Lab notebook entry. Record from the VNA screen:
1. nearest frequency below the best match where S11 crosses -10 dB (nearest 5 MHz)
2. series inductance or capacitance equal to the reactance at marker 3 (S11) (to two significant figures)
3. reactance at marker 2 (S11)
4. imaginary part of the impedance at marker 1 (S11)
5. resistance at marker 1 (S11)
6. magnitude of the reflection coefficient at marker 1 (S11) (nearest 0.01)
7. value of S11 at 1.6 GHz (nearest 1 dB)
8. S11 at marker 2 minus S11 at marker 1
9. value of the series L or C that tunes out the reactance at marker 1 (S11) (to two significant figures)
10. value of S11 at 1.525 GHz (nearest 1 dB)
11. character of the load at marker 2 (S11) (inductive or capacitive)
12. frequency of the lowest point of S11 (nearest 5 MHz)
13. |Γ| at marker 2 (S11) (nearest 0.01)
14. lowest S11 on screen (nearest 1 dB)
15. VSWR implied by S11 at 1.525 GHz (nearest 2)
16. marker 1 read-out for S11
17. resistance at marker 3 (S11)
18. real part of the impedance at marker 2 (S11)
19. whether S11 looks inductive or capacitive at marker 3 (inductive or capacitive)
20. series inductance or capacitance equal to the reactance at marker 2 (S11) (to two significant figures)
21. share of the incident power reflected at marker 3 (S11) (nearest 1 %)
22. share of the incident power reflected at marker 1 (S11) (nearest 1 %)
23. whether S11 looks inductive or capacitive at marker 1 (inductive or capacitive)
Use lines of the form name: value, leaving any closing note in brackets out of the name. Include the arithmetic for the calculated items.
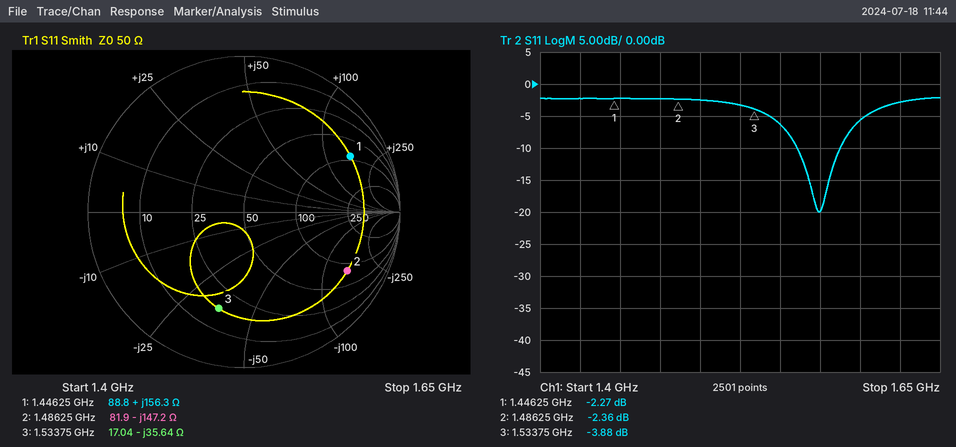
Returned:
nearest frequency below the best match where S11 crosses -10 dB: 1.560 GHz
series inductance or capacitance equal to the reactance at marker 3 (S11): C = 1/(2π × 1.53375 GHz × 35.64 Ω) ≈ 2.9 pF
reactance at marker 2: -147.2 Ω
imaginary part of the impedance at marker 1: +156.3 Ω
resistance at marker 1: 88.8 Ω
magnitude of the reflection coefficient at marker 1 (S11): 0.77
value of S11 at 1.6 GHz: -6 dB
S11 at marker 2 minus S11 at marker 1: -2.36 − (-2.27) = -0.09 dB
value of the series L or C that tunes out the reactance at marker 1 (S11): C = 1/(2π × 1.44625 GHz × 156.3 Ω) ≈ 704 fF, so 700 fF to two significant figures
value of S11 at 1.525 GHz: -3 dB
character of the load at marker 2 (S11): capacitive
frequency of the lowest point of S11: 1.575 GHz
|Γ| at marker 2 (S11): 0.76
lowest S11 on screen: -20 dB
VSWR implied by S11 at 1.525 GHz: |Γ| = 10^(-3/20) = 0.7079; VSWR = (1 + 0.7079)/(1 − 0.7079) ≈ 6
marker 1 read-out for S11: -2.27 dB
resistance at marker 3: 17.04 Ω
real part of the impedance at marker 2: 81.9 Ω
whether S11 looks inductive or capacitive at marker 3: capacitive
series inductance or capacitance equal to the reactance at marker 2 (S11): C = 1/(2π × 1.48625 GHz × 147.2 Ω) ≈ 727 fF, so 730 fF to two significant figures
share of the incident power reflected at marker 3 (S11): 10^(-3.88/10) ≈ 41 %
share of the incident power reflected at marker 1 (S11): 10^(-2.27/10) ≈ 59 %
whether S11 looks inductive or capacitive at marker 1: inductive
